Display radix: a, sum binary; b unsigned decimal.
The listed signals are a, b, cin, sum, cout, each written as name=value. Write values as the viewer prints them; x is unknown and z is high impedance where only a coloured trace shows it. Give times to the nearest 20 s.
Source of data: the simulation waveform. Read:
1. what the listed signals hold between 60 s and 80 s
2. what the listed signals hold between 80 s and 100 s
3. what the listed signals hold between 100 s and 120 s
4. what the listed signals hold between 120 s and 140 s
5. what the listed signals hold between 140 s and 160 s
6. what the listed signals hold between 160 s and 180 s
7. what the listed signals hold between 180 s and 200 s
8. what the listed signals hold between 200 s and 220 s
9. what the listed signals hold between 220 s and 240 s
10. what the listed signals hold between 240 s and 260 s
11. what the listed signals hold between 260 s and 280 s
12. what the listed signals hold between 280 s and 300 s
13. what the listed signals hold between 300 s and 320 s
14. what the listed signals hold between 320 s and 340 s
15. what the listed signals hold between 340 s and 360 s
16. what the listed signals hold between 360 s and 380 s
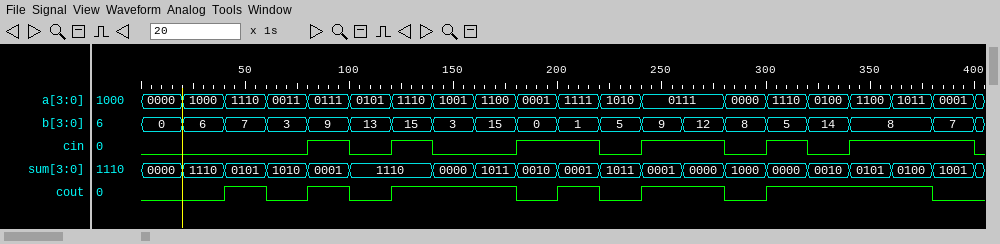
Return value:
a=0011, b=3, cin=0, sum=1010, cout=0
a=0111, b=9, cin=1, sum=0001, cout=1
a=0101, b=13, cin=0, sum=1110, cout=0
a=1110, b=15, cin=1, sum=1110, cout=1
a=1001, b=3, cin=0, sum=0000, cout=1
a=1100, b=15, cin=0, sum=1011, cout=1
a=0001, b=0, cin=1, sum=0010, cout=0
a=1111, b=1, cin=1, sum=0001, cout=1
a=1010, b=5, cin=0, sum=1011, cout=0
a=0111, b=9, cin=1, sum=0001, cout=1
a=0111, b=12, cin=1, sum=0000, cout=1
a=0000, b=8, cin=0, sum=1000, cout=0
a=1110, b=5, cin=1, sum=0000, cout=1
a=0100, b=14, cin=0, sum=0010, cout=1
a=1100, b=8, cin=1, sum=0101, cout=1
a=1011, b=8, cin=1, sum=0100, cout=1
